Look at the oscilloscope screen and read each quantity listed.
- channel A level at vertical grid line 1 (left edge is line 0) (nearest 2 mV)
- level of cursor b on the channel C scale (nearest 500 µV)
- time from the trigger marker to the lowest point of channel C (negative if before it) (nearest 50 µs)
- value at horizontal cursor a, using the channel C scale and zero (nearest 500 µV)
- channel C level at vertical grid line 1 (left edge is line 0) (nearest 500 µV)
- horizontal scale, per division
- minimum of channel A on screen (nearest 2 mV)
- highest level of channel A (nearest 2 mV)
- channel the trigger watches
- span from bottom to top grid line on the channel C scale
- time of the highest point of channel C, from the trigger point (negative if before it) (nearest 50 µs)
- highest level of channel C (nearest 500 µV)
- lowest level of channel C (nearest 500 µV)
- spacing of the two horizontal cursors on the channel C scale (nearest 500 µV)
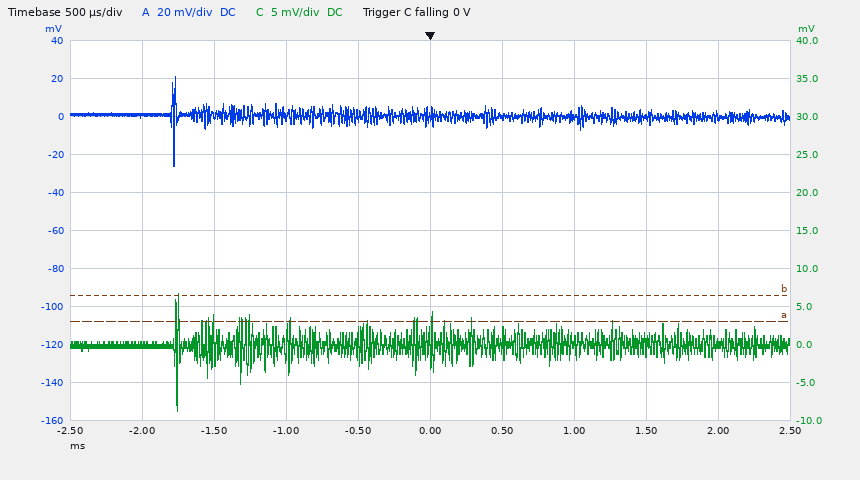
0 mV
6.5 mV
-1.75 ms
3.0 mV
0.0 mV
500 µs
-26 mV
22 mV
channel C
50 mV
-1.75 ms
6.5 mV
-8.5 mV
3.5 mV
